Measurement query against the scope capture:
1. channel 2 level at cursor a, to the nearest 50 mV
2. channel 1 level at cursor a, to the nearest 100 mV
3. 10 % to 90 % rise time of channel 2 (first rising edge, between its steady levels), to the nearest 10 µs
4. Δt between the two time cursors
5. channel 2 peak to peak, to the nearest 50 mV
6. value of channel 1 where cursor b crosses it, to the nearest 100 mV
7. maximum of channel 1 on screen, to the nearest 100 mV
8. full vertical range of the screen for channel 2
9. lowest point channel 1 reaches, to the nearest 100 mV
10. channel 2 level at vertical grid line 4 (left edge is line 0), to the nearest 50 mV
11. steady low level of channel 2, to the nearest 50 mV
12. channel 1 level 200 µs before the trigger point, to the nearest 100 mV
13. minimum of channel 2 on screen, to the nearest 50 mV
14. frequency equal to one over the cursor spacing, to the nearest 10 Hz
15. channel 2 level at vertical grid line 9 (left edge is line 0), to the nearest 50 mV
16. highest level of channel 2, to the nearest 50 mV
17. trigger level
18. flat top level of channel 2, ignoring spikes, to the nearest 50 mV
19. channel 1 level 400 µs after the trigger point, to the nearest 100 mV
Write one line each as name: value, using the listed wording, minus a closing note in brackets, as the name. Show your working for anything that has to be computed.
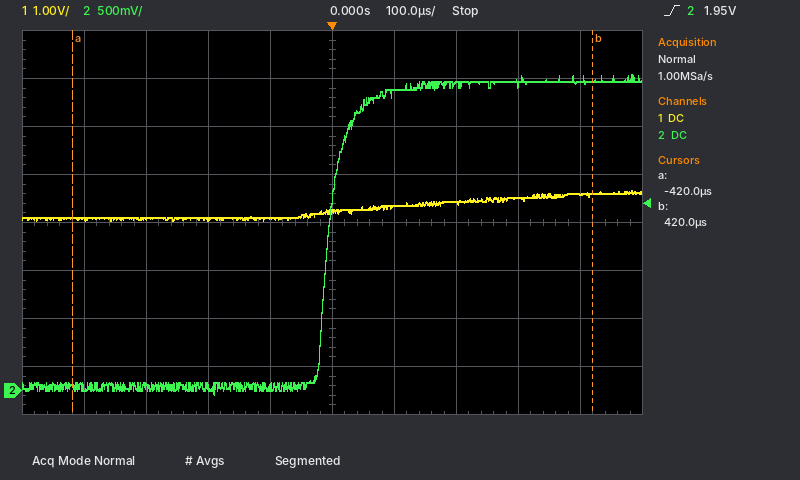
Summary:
channel 2 level at cursor a, to the nearest 50 mV: 50 mV
channel 1 level at cursor a, to the nearest 100 mV: 3.6 V
10 % to 90 % rise time of channel 2 (first rising edge, between its steady levels), to the nearest 10 µs: 60 µs
Δt between the two time cursors: 420 µs − (-420 µs) = 840 µs
channel 2 peak to peak, to the nearest 50 mV: 3.30 V − (-50 mV) = 3.35 V
value of channel 1 where cursor b crosses it, to the nearest 100 mV: 4.1 V
maximum of channel 1 on screen, to the nearest 100 mV: 4.2 V
full vertical range of the screen for channel 2: 4 V
lowest point channel 1 reaches, to the nearest 100 mV: 3.5 V
channel 2 level at vertical grid line 4 (left edge is line 0), to the nearest 50 mV: 50 mV
steady low level of channel 2, to the nearest 50 mV: 50 mV
channel 1 level 200 µs before the trigger point, to the nearest 100 mV: 3.6 V
minimum of channel 2 on screen, to the nearest 50 mV: -50 mV
frequency equal to one over the cursor spacing, to the nearest 10 Hz: 1 / 840 µs ≈ 1.19 kHz
channel 2 level at vertical grid line 9 (left edge is line 0), to the nearest 50 mV: 3.20 V
highest level of channel 2, to the nearest 50 mV: 3.30 V
trigger level: 1.95 V
flat top level of channel 2, ignoring spikes, to the nearest 50 mV: 3.20 V
channel 1 level 400 µs after the trigger point, to the nearest 100 mV: 4.1 V
